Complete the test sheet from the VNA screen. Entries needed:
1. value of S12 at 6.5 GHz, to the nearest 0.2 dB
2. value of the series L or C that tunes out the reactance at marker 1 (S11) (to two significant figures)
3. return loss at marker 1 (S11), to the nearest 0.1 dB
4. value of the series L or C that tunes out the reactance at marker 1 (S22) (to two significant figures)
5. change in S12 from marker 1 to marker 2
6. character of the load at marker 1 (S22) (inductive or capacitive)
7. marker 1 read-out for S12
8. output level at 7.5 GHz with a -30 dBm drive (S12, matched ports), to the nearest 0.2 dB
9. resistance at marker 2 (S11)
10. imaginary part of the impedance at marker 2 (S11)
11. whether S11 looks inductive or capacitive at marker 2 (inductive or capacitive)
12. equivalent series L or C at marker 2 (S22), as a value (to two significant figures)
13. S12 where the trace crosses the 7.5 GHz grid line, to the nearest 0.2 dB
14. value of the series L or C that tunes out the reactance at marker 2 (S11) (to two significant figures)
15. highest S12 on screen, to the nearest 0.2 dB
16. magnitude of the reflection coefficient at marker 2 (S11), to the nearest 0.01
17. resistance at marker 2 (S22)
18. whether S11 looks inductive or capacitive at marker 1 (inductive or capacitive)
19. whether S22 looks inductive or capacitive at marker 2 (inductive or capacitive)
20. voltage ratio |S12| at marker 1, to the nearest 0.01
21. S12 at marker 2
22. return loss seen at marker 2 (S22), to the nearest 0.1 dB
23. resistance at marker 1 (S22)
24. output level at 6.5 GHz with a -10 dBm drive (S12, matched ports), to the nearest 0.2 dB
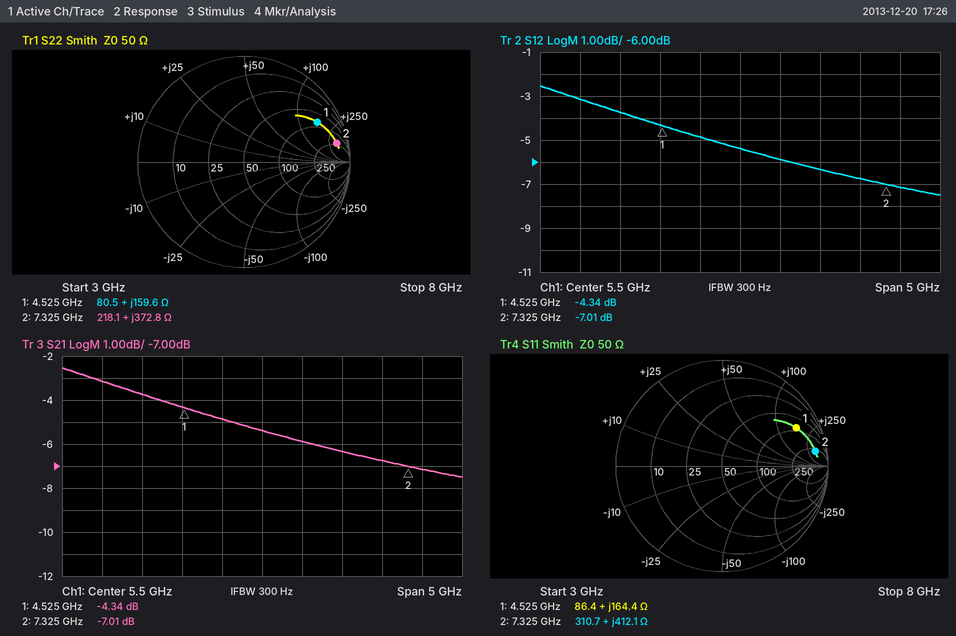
-6.4 dB
210 fF
2.1 dB
220 fF
-2.67 dB
inductive
-4.34 dB
-37.2 dBm
310.7 Ω
+412.1 Ω
inductive
8.1 nH
-7.2 dB
53 fF
-2.6 dB
0.89
218.1 Ω
inductive
inductive
0.61
-7.01 dB
1.0 dB
80.5 Ω
-16.4 dBm
